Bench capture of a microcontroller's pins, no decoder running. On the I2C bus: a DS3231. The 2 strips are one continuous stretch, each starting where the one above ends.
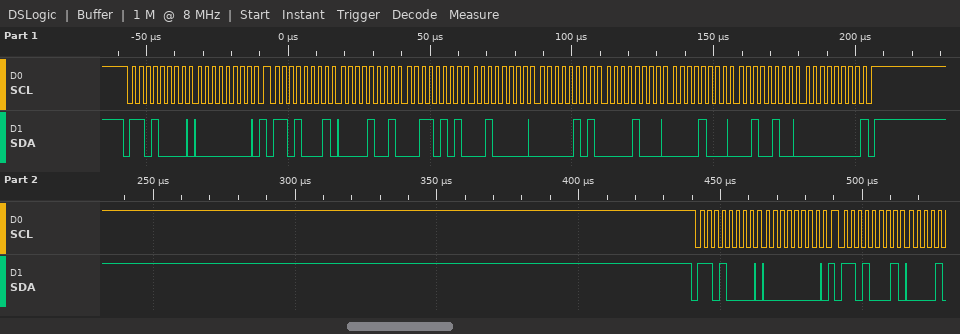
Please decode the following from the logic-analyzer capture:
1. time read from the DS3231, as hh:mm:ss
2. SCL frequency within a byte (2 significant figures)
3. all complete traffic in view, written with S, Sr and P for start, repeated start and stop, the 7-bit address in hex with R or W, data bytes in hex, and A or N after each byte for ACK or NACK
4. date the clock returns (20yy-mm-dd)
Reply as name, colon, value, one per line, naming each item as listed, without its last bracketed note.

time read from the DS3231, as hh:mm:ss: 20:35:09
SCL frequency within a byte: 400 kHz
all complete traffic in view, written with S, Sr and P for start, repeated start and stop, the 7-bit address in hex with R or W, data bytes in hex, and A or N after each byte for ACK or NACK: S 68W A 00 A Sr 68R A 09 A 35 A 20 A 05 A 08 A 08 A 24 A 00 N P S 68W A 00 A Sr 68R A
date the clock returns: 2024-08-08
